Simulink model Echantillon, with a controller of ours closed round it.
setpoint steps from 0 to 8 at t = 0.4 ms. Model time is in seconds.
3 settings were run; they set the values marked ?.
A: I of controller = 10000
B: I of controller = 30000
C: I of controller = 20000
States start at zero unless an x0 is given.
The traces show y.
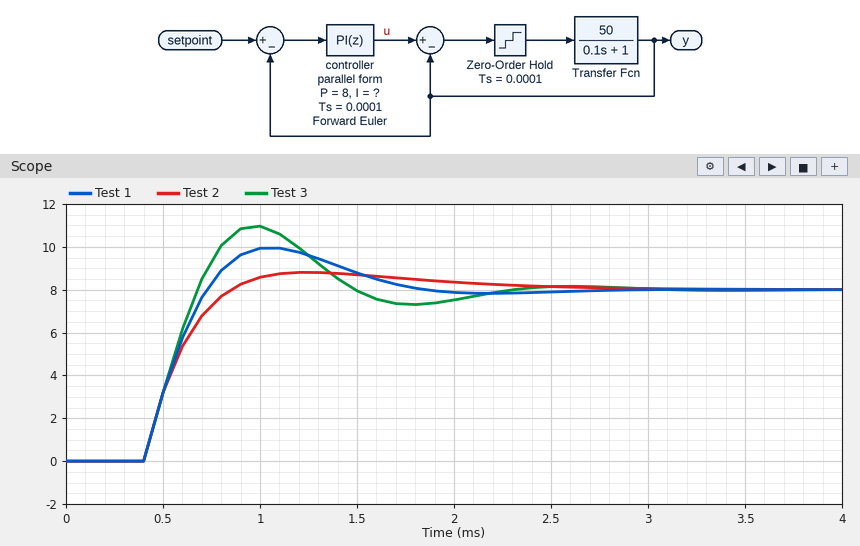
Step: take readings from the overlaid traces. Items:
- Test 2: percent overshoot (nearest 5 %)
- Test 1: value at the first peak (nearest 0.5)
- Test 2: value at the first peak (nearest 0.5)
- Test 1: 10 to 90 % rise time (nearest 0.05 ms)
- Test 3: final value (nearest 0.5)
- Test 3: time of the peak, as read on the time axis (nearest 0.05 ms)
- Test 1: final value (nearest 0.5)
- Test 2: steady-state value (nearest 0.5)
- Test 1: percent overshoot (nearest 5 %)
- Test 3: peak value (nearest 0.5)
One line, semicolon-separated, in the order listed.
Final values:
10 %; 10.0; 9.0; 0.25 ms; 8.0; 1.00 ms; 8.0; 8.0; 25 %; 11.0
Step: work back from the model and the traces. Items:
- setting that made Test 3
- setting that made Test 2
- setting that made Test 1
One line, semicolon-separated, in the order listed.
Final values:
B; A; C
